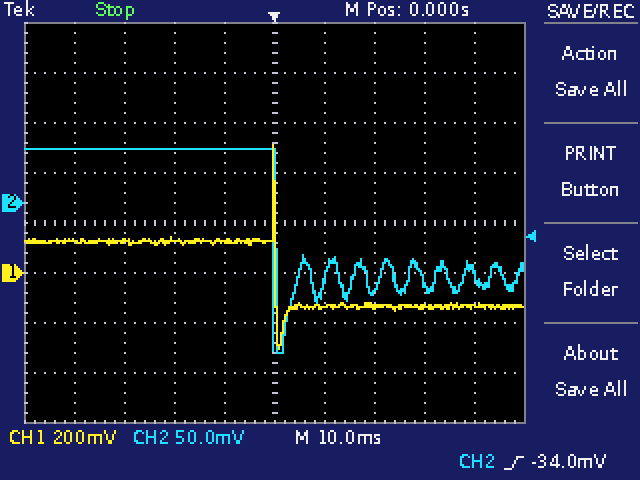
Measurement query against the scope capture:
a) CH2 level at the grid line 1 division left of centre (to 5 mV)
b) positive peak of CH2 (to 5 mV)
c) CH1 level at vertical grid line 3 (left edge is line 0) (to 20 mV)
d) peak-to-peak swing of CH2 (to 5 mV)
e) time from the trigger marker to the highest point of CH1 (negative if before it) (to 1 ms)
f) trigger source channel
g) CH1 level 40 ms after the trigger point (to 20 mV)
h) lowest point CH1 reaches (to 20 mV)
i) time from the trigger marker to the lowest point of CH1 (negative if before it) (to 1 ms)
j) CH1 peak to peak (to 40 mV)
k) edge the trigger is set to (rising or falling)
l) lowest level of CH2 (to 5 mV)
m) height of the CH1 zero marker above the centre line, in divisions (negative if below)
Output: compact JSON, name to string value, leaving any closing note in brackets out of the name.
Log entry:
{"CH2 level at the grid line 1 division left of centre": "55 mV", "positive peak of CH2": "55 mV", "CH1 level at vertical grid line 3 (left edge is line 0)": "140 mV", "peak-to-peak swing of CH2": "205 mV", "time from the trigger marker to the highest point of CH1 (negative if before it)": "0 ms", "trigger source channel": "CH2", "CH1 level 40 ms after the trigger point": "-140 mV", "lowest point CH1 reaches": "-300 mV", "time from the trigger marker to the lowest point of CH1 (negative if before it)": "+1 ms", "CH1 peak to peak": "800 mV", "edge the trigger is set to": "rising", "lowest level of CH2": "-150 mV", "height of the CH1 zero marker above the centre line, in divisions": "-1.0 div"}
